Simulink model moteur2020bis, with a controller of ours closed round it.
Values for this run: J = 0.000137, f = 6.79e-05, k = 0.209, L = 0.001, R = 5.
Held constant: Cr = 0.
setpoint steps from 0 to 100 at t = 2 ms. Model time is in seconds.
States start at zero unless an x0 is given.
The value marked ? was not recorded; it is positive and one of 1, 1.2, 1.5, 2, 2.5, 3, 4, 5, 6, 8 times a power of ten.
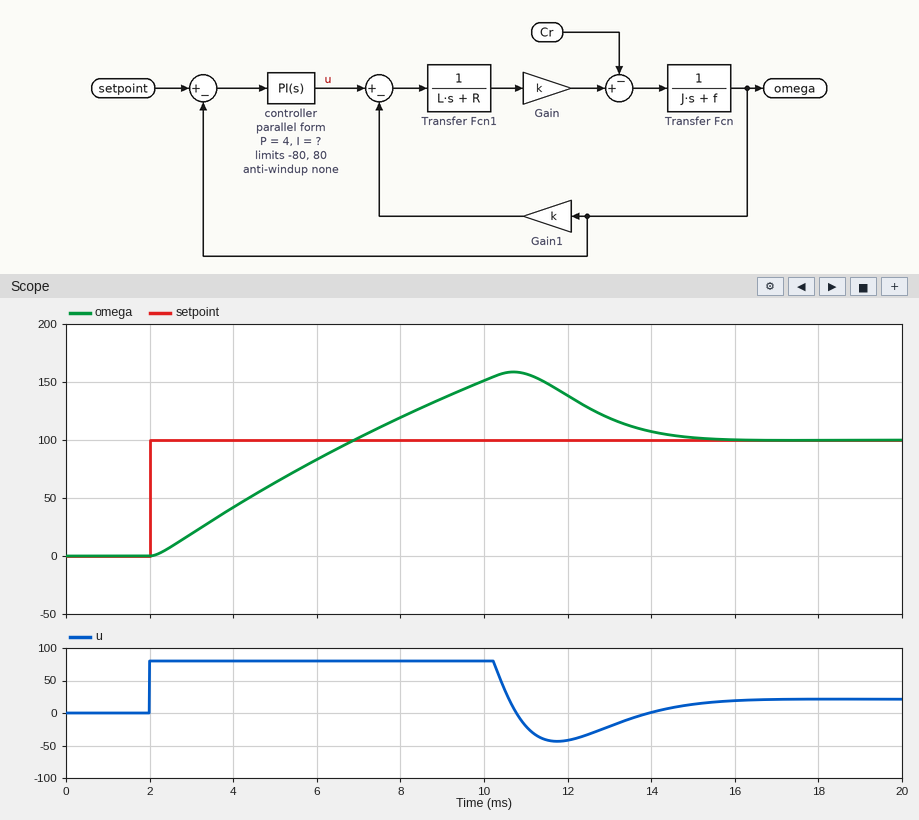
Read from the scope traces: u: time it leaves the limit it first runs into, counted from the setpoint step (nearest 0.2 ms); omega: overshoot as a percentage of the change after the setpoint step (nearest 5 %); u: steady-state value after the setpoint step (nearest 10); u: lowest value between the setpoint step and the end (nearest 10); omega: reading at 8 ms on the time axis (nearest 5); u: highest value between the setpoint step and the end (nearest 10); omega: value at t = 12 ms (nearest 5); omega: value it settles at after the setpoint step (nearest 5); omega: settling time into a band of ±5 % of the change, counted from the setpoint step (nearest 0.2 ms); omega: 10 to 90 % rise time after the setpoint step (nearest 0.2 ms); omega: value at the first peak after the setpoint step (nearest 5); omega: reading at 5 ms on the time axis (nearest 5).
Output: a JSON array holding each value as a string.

["8.2 ms", "60 %", "20", "-40", "120", "80", "140", "100", "12.4 ms", "3.8 ms", "160", "65"]
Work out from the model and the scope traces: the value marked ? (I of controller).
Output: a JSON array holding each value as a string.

["2000"]
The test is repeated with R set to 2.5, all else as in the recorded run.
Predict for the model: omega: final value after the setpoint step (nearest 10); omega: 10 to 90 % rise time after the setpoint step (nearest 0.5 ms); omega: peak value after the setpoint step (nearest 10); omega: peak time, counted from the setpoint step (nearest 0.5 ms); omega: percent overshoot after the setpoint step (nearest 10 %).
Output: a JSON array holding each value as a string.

["100", "2.0 ms", "150", "4.5 ms", "50 %"]
